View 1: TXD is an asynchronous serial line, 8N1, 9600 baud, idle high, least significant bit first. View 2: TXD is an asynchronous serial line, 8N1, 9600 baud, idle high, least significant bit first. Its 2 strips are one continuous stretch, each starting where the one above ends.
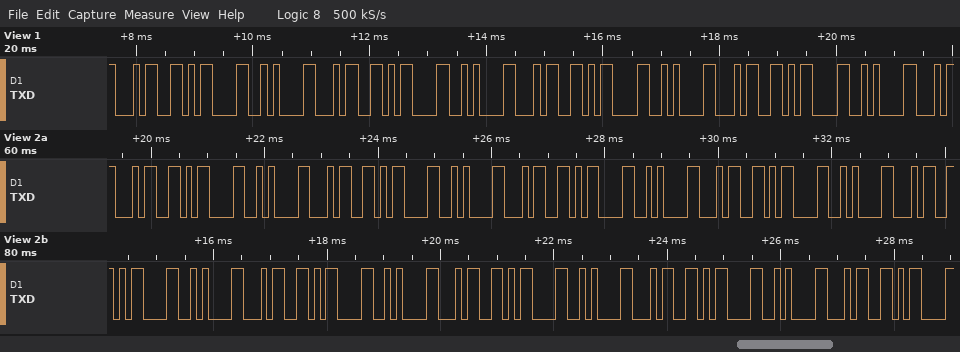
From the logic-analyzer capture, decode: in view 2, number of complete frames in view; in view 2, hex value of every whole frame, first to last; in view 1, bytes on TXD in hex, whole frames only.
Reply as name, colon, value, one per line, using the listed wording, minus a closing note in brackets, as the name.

in view 2, number of complete frames in view: 26
in view 2, hex value of every whole frame, first to last: 34 0D 0A 34 0D 0A 34 0D 0A 34 0D 0A 34 0D 0A 34 0D 0A 34 0D 0A 34 0D 0A 34 0D
in view 1, bytes on TXD in hex, whole frames only: 34 0D 0A 34 0D 0A 34 0D 0A 34 0D 0A
